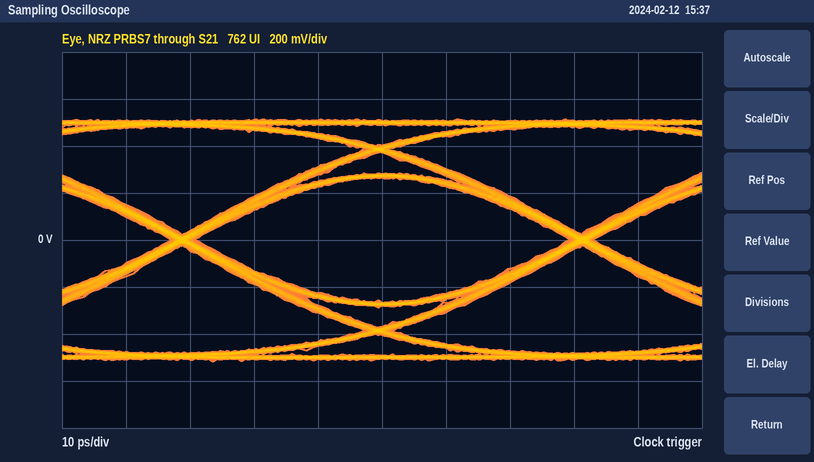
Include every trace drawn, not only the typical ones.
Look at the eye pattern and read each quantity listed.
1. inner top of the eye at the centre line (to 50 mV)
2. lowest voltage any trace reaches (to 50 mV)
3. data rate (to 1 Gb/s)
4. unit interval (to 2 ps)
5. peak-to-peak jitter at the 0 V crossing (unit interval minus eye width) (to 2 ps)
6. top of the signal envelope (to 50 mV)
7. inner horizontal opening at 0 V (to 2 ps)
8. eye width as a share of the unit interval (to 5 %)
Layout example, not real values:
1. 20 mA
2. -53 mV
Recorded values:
1. 250 mV
2. -500 mV
3. 16 Gb/s
4. 62 ps
5. 4 ps
6. 500 mV
7. 58 ps
8. 95 %
